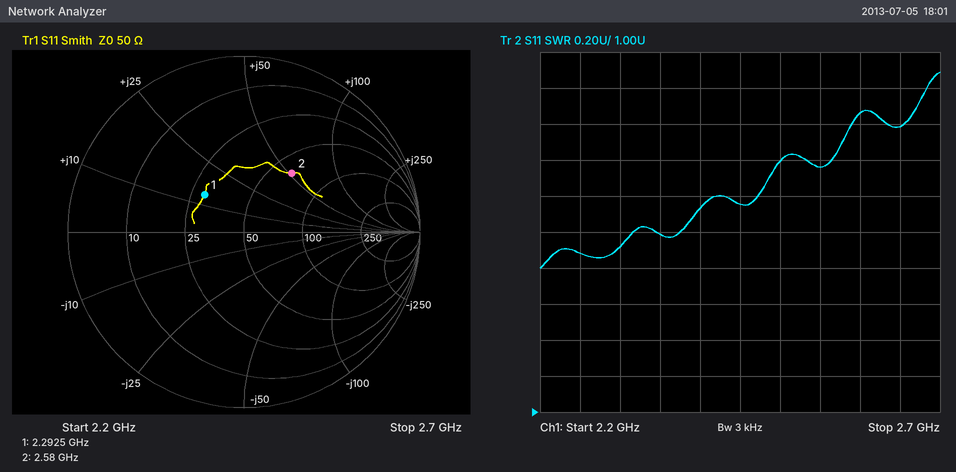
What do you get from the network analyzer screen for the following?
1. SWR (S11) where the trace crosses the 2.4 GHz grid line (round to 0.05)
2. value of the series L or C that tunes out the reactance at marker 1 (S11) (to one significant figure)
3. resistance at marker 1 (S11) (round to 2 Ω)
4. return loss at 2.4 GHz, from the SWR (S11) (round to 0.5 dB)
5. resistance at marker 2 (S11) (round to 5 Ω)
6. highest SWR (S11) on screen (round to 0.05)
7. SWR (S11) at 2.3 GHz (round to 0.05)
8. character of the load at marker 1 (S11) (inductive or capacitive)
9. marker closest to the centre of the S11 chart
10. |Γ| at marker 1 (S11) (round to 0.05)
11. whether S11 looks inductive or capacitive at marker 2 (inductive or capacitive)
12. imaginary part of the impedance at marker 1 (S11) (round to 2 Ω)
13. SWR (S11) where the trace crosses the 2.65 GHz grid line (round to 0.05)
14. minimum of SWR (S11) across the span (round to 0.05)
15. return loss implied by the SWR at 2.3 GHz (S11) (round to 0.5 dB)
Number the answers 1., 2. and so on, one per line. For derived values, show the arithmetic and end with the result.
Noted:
1. 2.15
2. C = 1/(2π × 2.2925 GHz × 14 Ω) ≈ 5 pF
3. 30 Ω
4. −20 log10((2.15 − 1)/(2.15 + 1)) ≈ 8.75 dB, so 9.0 dB to the nearest 0.5 dB
5. 65 Ω
6. 2.90
7. 1.90
8. inductive
9. marker 1
10. 0.30
11. inductive
12. +14 Ω
13. 2.60
14. 1.80
15. −20 log10((1.9 − 1)/(1.9 + 1)) ≈ 10.2 dB, so 10.0 dB to the nearest 0.5 dB
